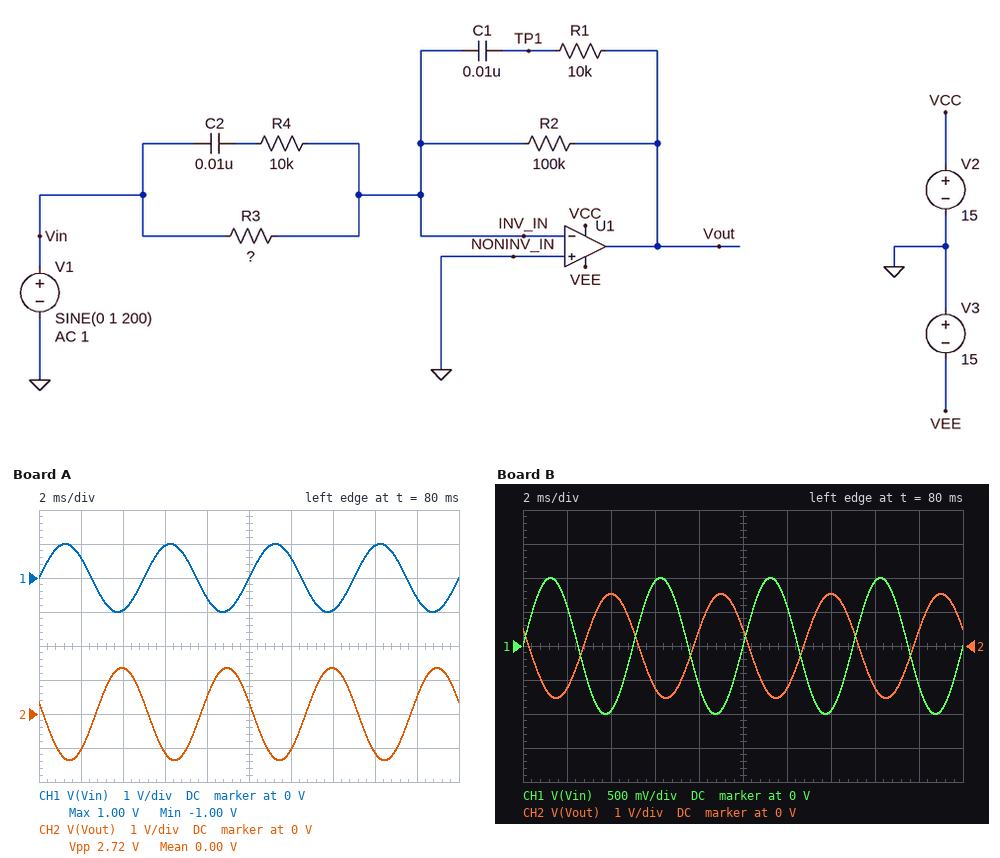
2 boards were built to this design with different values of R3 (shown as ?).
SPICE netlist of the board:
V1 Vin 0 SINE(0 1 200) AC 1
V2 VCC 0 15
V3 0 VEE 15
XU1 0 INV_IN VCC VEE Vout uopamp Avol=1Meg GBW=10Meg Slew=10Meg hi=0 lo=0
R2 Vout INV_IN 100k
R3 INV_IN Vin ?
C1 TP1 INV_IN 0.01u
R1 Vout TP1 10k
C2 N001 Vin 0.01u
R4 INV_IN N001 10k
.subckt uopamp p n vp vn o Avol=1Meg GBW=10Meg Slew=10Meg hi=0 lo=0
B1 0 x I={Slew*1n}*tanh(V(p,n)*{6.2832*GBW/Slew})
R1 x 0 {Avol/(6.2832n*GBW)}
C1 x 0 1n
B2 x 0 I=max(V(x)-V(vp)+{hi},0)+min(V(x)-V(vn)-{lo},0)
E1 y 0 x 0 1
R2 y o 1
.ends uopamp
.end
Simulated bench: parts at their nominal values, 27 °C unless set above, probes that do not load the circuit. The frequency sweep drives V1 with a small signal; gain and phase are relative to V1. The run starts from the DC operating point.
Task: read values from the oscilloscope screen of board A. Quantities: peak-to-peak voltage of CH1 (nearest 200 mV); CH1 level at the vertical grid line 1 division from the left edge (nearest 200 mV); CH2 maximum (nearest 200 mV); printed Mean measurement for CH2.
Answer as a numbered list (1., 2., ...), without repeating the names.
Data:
1. 2.0 V
2. 600 mV
3. 1.4 V
4. 0.00 V
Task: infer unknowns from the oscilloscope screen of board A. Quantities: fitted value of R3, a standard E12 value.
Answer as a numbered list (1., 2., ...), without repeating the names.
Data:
1. 56 kΩ
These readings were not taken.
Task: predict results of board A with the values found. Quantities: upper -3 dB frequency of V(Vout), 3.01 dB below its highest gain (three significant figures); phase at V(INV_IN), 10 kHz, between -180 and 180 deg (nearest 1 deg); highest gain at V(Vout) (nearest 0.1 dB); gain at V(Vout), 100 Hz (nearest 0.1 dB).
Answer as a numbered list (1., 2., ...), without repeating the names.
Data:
1. 273 Hz
2. 89 deg
3. 5.0 dB
4. 4.0 dB
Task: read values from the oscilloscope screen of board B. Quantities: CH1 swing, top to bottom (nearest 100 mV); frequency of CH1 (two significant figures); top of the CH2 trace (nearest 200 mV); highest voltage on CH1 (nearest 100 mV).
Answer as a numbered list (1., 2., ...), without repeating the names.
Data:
1. 2.0 V
2. 200 Hz
3. 1.6 V
4. 1.0 V
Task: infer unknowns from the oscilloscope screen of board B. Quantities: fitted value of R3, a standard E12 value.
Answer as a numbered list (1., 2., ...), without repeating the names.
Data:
1. 47 kΩ
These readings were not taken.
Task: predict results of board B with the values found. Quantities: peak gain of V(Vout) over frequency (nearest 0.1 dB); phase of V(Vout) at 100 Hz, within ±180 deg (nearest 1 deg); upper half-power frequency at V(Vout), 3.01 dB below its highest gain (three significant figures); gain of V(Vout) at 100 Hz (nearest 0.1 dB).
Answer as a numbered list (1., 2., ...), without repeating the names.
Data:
1. 6.6 dB
2. 165 deg
3. 213 Hz
4. 5.4 dB
